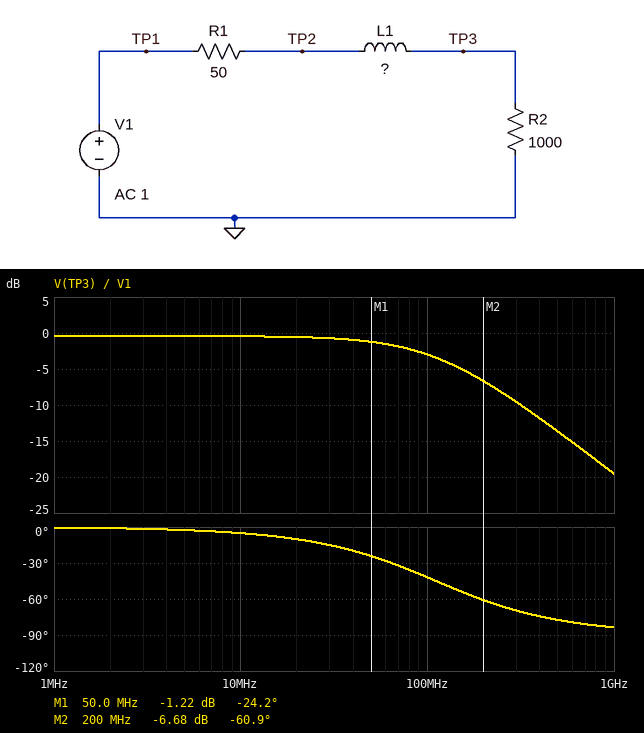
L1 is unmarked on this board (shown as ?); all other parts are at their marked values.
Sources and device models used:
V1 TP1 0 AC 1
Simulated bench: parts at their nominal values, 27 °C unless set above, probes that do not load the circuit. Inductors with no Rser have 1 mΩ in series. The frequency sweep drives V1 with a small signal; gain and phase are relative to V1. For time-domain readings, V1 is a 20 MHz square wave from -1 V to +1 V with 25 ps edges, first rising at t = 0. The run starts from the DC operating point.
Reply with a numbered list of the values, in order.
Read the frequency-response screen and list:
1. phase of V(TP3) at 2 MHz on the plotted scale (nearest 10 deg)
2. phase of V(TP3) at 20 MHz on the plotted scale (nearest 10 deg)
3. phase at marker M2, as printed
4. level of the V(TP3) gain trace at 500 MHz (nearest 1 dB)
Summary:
1. 0 deg
2. -10 deg
3. -60.9 deg
4. -14 dB
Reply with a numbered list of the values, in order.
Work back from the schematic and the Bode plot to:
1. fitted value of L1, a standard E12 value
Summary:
1. 1.5 µH
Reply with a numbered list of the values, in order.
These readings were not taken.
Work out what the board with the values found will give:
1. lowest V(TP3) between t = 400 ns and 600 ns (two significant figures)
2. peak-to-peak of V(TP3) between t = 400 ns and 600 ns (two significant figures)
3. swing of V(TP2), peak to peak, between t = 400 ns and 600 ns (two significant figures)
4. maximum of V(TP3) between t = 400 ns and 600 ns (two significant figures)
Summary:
1. -950 mV
2. 1.9 V
3. 2.1 V
4. 950 mV
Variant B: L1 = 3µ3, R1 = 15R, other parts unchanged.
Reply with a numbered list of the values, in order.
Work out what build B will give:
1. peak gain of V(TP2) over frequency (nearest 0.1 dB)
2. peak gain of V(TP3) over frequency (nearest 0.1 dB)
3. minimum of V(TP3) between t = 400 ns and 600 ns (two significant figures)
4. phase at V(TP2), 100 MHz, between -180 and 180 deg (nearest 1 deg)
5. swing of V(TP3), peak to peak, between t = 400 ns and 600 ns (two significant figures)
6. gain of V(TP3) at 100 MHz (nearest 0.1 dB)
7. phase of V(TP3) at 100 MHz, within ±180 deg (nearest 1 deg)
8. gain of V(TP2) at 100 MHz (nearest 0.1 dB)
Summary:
1. 0 dB
2. -0.1 dB
3. -980 mV
4. 0 deg
5. 2.0 V
6. -7.3 dB
7. -64 deg
8. 0 dB
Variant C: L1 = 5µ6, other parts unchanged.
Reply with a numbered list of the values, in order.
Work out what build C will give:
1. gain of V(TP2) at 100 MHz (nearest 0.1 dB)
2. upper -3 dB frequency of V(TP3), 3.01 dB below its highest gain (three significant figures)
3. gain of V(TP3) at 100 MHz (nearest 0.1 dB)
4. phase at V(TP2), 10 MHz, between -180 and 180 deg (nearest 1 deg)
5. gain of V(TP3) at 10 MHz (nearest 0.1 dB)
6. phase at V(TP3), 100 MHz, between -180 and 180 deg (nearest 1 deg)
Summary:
1. 0 dB
2. 29.8 MHz
3. -11.3 dB
4. 1 deg
5. -0.9 dB
6. -73 deg
